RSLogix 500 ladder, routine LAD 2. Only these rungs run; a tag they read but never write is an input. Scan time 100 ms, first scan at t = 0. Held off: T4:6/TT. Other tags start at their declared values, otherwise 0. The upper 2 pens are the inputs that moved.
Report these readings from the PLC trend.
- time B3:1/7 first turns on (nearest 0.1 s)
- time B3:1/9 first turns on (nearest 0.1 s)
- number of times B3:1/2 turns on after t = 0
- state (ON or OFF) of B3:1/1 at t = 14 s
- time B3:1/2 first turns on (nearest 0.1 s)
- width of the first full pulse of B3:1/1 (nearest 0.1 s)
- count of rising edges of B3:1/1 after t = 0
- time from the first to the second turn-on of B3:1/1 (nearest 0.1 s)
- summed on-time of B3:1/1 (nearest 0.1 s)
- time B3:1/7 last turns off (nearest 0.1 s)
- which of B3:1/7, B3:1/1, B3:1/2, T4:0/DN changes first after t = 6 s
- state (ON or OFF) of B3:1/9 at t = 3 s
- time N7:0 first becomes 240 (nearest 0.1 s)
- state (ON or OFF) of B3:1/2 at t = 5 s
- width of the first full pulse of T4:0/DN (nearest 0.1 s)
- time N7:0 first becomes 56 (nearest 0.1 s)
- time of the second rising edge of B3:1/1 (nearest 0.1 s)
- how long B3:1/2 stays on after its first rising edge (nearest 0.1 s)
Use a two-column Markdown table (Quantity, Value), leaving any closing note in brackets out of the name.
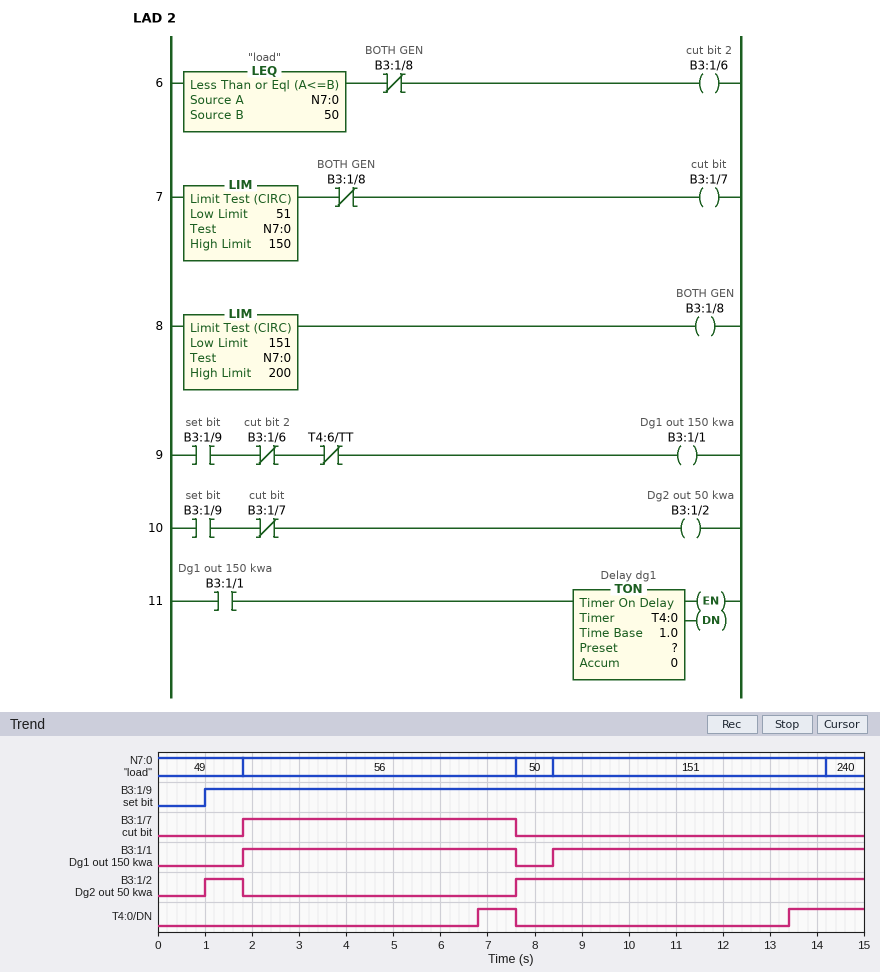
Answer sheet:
| Quantity | Value |
|---|---|
| time B3:1/7 first turns on | 1.8 s |
| time B3:1/9 first turns on | 1.0 s |
| number of times B3:1/2 turns on after t = 0 | 2 |
| state (ON or OFF) of B3:1/1 at t = 14 s | ON |
| time B3:1/2 first turns on | 1.0 s |
| width of the first full pulse of B3:1/1 | 5.8 s |
| count of rising edges of B3:1/1 after t = 0 | 2 |
| time from the first to the second turn-on of B3:1/1 | 6.6 s |
| summed on-time of B3:1/1 | 12.4 s |
| time B3:1/7 last turns off | 7.6 s |
| which of B3:1/7, B3:1/1, B3:1/2, T4:0/DN changes first after t = 6 s | T4:0/DN |
| state (ON or OFF) of B3:1/9 at t = 3 s | ON |
| time N7:0 first becomes 240 | 14.2 s |
| state (ON or OFF) of B3:1/2 at t = 5 s | OFF |
| width of the first full pulse of T4:0/DN | 0.8 s |
| time N7:0 first becomes 56 | 1.8 s |
| time of the second rising edge of B3:1/1 | 8.4 s |
| how long B3:1/2 stays on after its first rising edge | 0.8 s |
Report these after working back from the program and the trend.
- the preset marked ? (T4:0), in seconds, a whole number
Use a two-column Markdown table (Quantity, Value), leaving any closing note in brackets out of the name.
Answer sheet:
| Quantity | Value |
|---|---|
| the preset marked ? (T4:0), in seconds, a whole number | 5 s |
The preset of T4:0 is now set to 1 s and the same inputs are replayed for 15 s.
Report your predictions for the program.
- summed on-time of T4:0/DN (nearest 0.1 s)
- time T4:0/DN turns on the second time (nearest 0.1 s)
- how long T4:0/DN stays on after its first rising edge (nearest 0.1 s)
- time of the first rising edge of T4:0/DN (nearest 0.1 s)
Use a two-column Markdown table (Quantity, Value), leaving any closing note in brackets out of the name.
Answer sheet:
| Quantity | Value |
|---|---|
| summed on-time of T4:0/DN | 10.4 s |
| time T4:0/DN turns on the second time | 9.4 s |
| how long T4:0/DN stays on after its first rising edge | 4.8 s |
| time of the first rising edge of T4:0/DN | 2.8 s |
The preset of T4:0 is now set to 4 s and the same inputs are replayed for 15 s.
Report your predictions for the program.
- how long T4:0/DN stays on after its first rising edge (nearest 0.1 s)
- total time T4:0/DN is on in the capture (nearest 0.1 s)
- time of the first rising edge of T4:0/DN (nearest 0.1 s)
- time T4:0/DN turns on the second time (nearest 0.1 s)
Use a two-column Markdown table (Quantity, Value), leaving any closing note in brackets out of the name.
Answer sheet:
| Quantity | Value |
|---|---|
| how long T4:0/DN stays on after its first rising edge | 1.8 s |
| total time T4:0/DN is on in the capture | 4.4 s |
| time of the first rising edge of T4:0/DN | 5.8 s |
| time T4:0/DN turns on the second time | 12.4 s |
